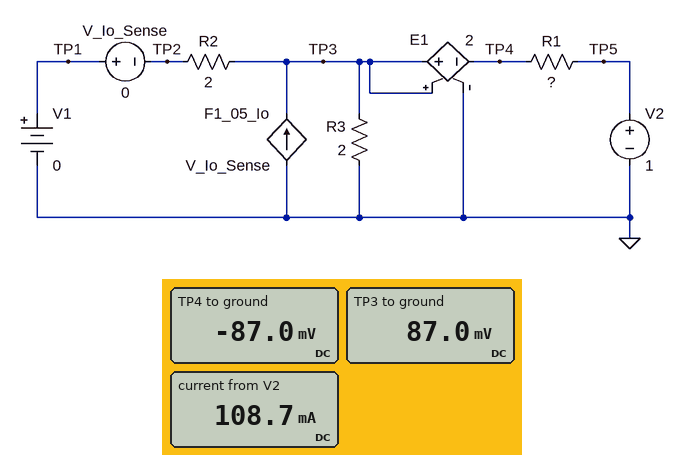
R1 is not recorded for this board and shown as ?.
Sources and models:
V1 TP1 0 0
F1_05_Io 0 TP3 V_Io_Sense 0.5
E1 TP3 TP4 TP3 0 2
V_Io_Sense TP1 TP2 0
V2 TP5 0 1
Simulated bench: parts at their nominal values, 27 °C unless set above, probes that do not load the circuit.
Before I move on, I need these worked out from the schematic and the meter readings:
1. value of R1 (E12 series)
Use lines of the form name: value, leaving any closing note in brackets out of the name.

value of R1: 10 Ω
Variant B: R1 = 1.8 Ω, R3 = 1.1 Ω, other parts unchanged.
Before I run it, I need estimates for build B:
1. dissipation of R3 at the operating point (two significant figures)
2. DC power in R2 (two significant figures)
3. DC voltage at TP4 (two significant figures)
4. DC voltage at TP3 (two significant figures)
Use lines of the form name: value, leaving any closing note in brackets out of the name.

dissipation of R3 at the operating point: 230 mW
DC power in R2: 130 mW
DC voltage at TP4: -500 mV
DC voltage at TP3: 500 mV
